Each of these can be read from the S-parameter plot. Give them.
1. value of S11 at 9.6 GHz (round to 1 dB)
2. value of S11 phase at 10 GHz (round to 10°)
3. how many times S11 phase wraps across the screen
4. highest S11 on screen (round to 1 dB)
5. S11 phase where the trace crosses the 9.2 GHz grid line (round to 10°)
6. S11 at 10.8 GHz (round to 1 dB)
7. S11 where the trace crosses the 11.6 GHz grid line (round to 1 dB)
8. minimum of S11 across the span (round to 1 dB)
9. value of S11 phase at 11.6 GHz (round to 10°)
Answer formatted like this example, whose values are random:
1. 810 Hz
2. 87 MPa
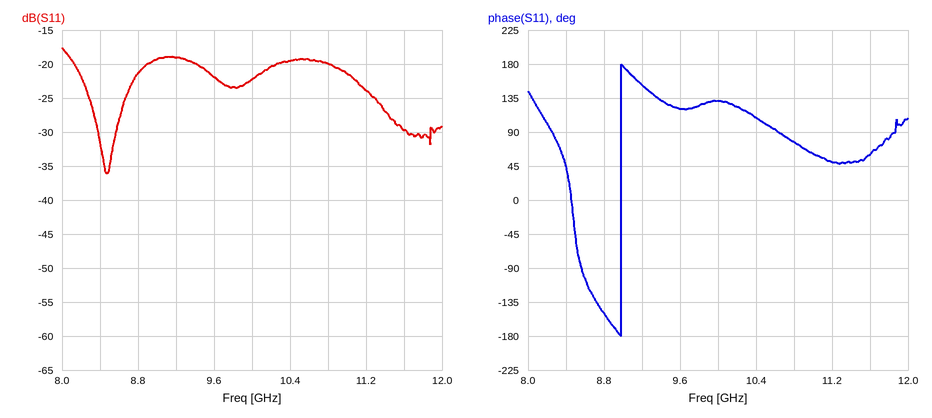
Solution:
1. -22 dB
2. 130°
3. 1
4. -18 dB
5. 150°
6. -20 dB
7. -30 dB
8. -36 dB
9. 60°
